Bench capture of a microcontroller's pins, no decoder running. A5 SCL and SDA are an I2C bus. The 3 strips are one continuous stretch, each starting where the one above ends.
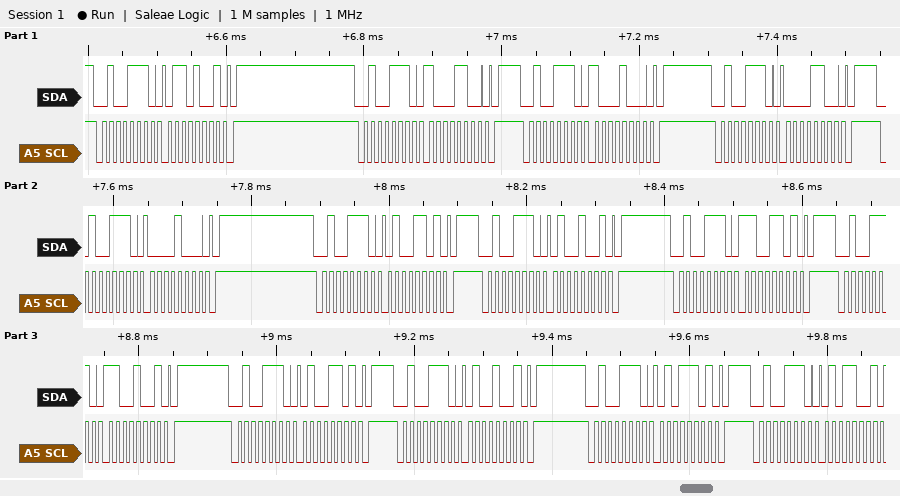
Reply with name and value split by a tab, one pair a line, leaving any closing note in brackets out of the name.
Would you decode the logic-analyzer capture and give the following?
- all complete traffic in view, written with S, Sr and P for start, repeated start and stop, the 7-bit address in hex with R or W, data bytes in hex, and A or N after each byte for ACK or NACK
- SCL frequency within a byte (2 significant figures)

all complete traffic in view, written with S, Sr and P for start, repeated start and stop, the 7-bit address in hex with R or W, data bytes in hex, and A or N after each byte for ACK or NACK	S 27W A 69 A P S 27W A 8C A P S 27W A 88 A P S 27W A 0C A P S 27W A 08 A P S 27W A 4D A P S 27W A 49 A P S 27W A CD A P S 27W A C9 A P S 27W A 4D A P S 27W A 49 A P S 27W A 5D A P S 27W A 59 A
SCL frequency within a byte	100 kHz
